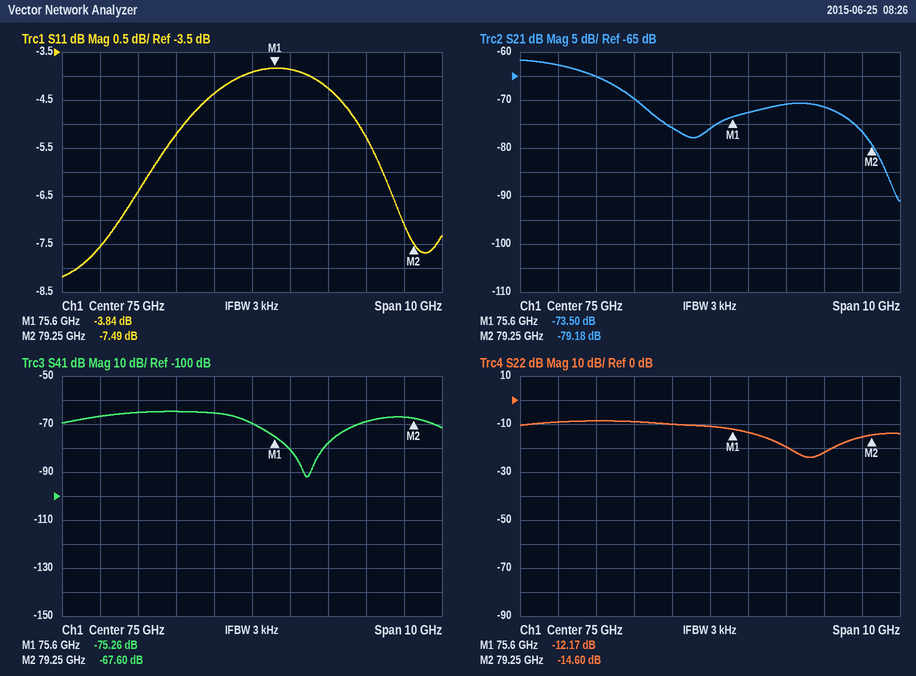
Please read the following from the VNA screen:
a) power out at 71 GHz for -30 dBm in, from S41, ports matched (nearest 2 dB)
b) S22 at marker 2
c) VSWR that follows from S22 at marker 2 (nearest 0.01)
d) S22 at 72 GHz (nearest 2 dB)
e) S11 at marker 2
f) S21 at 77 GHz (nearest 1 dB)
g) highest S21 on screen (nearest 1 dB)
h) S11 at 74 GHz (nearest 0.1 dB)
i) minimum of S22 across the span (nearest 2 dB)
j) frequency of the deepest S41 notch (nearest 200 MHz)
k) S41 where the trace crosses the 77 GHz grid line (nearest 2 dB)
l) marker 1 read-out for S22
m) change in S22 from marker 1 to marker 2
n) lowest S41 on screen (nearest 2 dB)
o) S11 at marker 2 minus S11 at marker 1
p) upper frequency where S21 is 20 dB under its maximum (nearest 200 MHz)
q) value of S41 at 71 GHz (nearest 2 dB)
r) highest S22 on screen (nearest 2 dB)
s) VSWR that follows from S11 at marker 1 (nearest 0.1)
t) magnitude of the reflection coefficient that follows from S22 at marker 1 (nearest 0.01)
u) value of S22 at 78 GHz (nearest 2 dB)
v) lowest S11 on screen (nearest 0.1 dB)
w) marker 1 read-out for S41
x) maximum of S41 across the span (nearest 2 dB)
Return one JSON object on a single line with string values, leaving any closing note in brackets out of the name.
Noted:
{"power out at 71 GHz for -30 dBm in, from S41, ports matched": "-96 dBm", "S22 at marker 2": "-14.60 dB", "VSWR that follows from S22 at marker 2": "1.46", "S22 at 72 GHz": "-8 dB", "S11 at marker 2": "-7.49 dB", "S21 at 77 GHz": "-71 dB", "highest S21 on screen": "-62 dB", "S11 at 74 GHz": "-4.4 dB", "minimum of S22 across the span": "-24 dB", "frequency of the deepest S41 notch": "76.4 GHz", "S41 where the trace crosses the 77 GHz grid line": "-78 dB", "marker 1 read-out for S22": "-12.17 dB", "change in S22 from marker 1 to marker 2": "-2.43 dB", "lowest S41 on screen": "-92 dB", "S11 at marker 2 minus S11 at marker 1": "-3.65 dB", "upper frequency where S21 is 20 dB under its maximum": "79.4 GHz", "value of S41 at 71 GHz": "-66 dB", "highest S22 on screen": "-8 dB", "VSWR that follows from S11 at marker 1": "4.6", "magnitude of the reflection coefficient that follows from S22 at marker 1": "0.25", "value of S22 at 78 GHz": "-22 dB", "lowest S11 on screen": "-8.2 dB", "marker 1 read-out for S41": "-75.26 dB", "maximum of S41 across the span": "-64 dB"}
